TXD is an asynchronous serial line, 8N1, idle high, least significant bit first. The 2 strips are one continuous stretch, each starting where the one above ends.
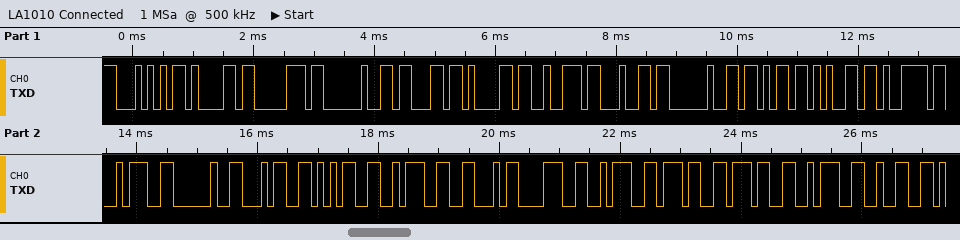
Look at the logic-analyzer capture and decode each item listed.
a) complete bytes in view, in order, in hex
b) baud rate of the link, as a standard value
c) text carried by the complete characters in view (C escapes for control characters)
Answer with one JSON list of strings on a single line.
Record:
["54 61 70 20 63 61 72 64 20 6B 65 79 3A 20 34 35 3A 46 38 3A 37 37 3A 32", "9600 baud", "\"Tap card key: 45:F8:77:2\""]
